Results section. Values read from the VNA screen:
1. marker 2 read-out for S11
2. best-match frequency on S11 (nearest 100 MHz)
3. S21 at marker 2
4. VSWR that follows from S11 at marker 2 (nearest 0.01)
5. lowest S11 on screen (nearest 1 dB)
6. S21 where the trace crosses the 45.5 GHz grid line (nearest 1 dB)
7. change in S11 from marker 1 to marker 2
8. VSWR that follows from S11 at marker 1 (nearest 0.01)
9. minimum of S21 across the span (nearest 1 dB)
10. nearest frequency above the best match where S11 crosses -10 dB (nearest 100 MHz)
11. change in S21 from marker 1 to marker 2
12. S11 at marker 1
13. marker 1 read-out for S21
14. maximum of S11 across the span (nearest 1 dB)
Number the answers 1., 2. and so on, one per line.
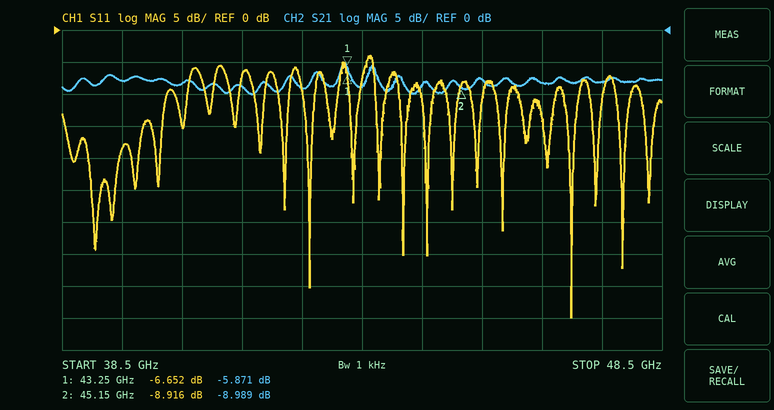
1. -8.916 dB
2. 47.0 GHz
3. -8.989 dB
4. 2.12
5. -45 dB
6. -8 dB
7. -2.264 dB
8. 2.74
9. -10 dB
10. 47.1 GHz
11. -3.118 dB
12. -6.652 dB
13. -5.871 dB
14. -4 dB
